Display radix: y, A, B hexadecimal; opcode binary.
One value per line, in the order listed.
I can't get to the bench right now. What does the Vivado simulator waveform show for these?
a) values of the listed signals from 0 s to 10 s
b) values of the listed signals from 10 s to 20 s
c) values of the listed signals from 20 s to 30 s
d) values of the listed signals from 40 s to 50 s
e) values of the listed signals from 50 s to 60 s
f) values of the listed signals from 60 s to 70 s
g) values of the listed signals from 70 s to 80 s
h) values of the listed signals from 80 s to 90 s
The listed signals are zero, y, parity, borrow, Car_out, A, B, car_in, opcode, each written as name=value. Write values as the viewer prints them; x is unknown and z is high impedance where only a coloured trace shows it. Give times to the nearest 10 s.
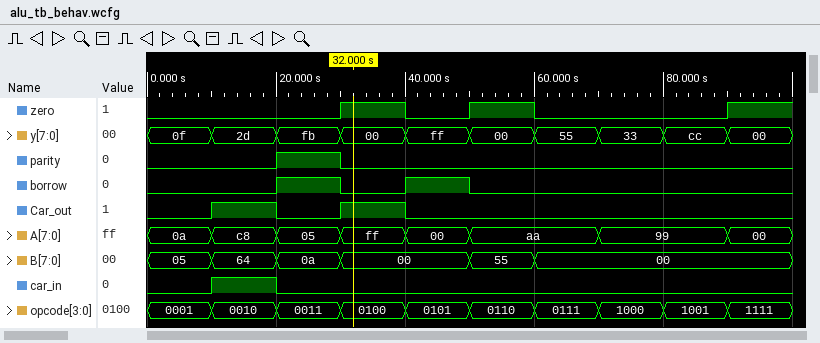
zero=0, y=0f, parity=0, borrow=0, Car_out=0, A=0a, B=05, car_in=0, opcode=0001
zero=0, y=2d, parity=0, borrow=0, Car_out=1, A=c8, B=64, car_in=1, opcode=0010
zero=0, y=fb, parity=1, borrow=1, Car_out=0, A=05, B=0a, car_in=0, opcode=0011
zero=0, y=ff, parity=0, borrow=1, Car_out=0, A=00, B=00, car_in=0, opcode=0101
zero=1, y=00, parity=0, borrow=0, Car_out=0, A=aa, B=55, car_in=0, opcode=0110
zero=0, y=55, parity=0, borrow=0, Car_out=0, A=aa, B=00, car_in=0, opcode=0111
zero=0, y=33, parity=0, borrow=0, Car_out=0, A=99, B=00, car_in=0, opcode=1000
zero=0, y=cc, parity=0, borrow=0, Car_out=0, A=99, B=00, car_in=0, opcode=1001
